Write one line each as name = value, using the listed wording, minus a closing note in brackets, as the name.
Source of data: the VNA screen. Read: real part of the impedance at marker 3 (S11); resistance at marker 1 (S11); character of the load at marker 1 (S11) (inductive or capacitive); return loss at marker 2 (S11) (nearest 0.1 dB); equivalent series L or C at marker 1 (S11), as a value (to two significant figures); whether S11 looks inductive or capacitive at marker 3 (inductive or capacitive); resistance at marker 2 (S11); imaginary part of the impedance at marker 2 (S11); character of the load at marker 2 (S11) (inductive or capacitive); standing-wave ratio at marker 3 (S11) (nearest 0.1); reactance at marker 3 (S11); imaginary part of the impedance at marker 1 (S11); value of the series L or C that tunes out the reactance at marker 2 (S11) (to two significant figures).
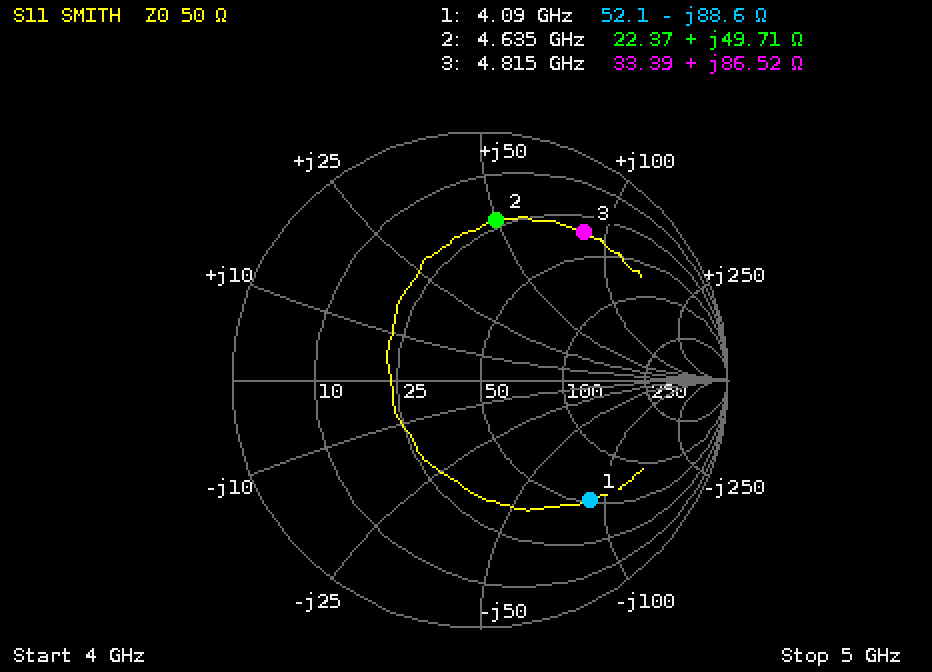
real part of the impedance at marker 3 = 33.39 Ω
resistance at marker 1 = 52.1 Ω
character of the load at marker 1 (S11) = capacitive
return loss at marker 2 (S11) = 3.8 dB
equivalent series L or C at marker 1 (S11), as a value = 440 fF
whether S11 looks inductive or capacitive at marker 3 = inductive
resistance at marker 2 = 22.37 Ω
imaginary part of the impedance at marker 2 = +49.71 Ω
character of the load at marker 2 (S11) = inductive
standing-wave ratio at marker 3 (S11) = 6.5
reactance at marker 3 = +86.52 Ω
imaginary part of the impedance at marker 1 = -88.6 Ω
value of the series L or C that tunes out the reactance at marker 2 (S11) = 690 fF
